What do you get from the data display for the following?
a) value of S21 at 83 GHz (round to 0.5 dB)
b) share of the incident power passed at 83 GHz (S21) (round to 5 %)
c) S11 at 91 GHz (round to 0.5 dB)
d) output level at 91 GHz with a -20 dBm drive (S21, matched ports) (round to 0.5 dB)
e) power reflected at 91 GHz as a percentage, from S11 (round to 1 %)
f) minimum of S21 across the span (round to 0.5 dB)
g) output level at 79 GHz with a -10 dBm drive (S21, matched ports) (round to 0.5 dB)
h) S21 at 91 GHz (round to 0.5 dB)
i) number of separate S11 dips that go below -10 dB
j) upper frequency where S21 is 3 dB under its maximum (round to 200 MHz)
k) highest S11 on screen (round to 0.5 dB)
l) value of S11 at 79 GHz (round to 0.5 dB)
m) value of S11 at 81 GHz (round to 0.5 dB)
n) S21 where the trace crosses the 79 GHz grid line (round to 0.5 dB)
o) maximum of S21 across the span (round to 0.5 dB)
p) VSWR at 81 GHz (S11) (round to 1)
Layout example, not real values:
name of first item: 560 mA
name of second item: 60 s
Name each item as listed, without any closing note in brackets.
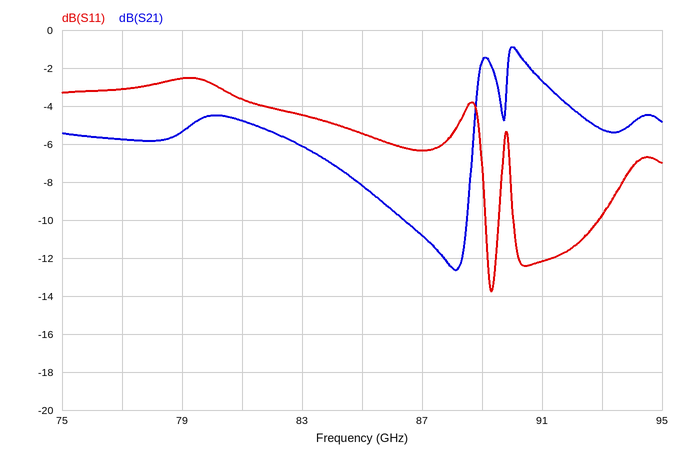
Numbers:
value of S21 at 83 GHz: -6.0 dB
share of the incident power passed at 83 GHz (S21): 25 %
S11 at 91 GHz: -12.0 dB
output level at 91 GHz with a -20 dBm drive (S21, matched ports): -22.5 dBm
power reflected at 91 GHz as a percentage, from S11: 6 %
minimum of S21 across the span: -12.5 dB
output level at 79 GHz with a -10 dBm drive (S21, matched ports): -15.5 dBm
S21 at 91 GHz: -2.5 dB
number of separate S11 dips that go below -10 dB: 2
upper frequency where S21 is 3 dB under its maximum: 91.8 GHz
highest S11 on screen: -2.5 dB
value of S11 at 79 GHz: -2.5 dB
value of S11 at 81 GHz: -3.5 dB
S21 where the trace crosses the 79 GHz grid line: -5.5 dB
maximum of S21 across the span: -1.0 dB
VSWR at 81 GHz (S11): 5
